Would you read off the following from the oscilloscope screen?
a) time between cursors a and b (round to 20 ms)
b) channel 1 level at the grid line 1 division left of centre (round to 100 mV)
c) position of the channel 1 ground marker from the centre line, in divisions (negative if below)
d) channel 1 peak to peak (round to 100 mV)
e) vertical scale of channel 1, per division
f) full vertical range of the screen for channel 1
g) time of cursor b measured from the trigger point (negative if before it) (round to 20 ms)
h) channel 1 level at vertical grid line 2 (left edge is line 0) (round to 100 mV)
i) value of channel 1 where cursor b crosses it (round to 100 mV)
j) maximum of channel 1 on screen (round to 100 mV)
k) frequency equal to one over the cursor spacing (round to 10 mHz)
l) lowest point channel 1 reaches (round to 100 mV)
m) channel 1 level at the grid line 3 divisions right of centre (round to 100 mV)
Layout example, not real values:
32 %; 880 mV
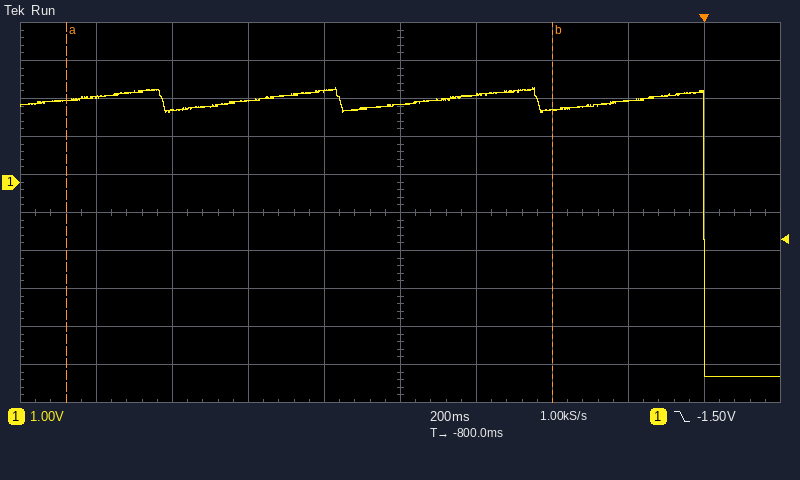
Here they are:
1.28 s; 2.4 V; +0.8 div; 7.6 V; 1 V; 10 V; -400 ms; 1.9 V; 1.9 V; 2.5 V; 780 mHz; -5.1 V; 2.1 V
